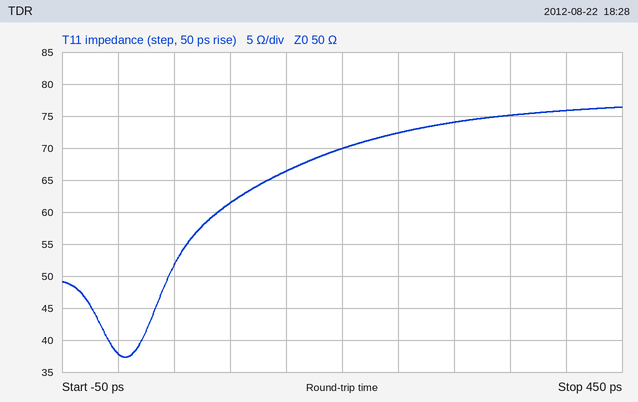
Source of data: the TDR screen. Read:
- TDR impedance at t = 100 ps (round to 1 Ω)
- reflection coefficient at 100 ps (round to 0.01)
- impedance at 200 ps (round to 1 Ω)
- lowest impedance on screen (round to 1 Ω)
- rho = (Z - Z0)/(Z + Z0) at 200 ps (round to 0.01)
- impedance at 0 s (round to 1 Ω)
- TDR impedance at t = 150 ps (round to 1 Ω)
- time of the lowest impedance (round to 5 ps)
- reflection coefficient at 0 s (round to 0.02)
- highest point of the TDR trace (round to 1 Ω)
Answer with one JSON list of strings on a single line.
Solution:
["61 Ω", "+0.10", "70 Ω", "37 Ω", "+0.17", "38 Ω", "66 Ω", "5 ps", "-0.14", "76 Ω"]
